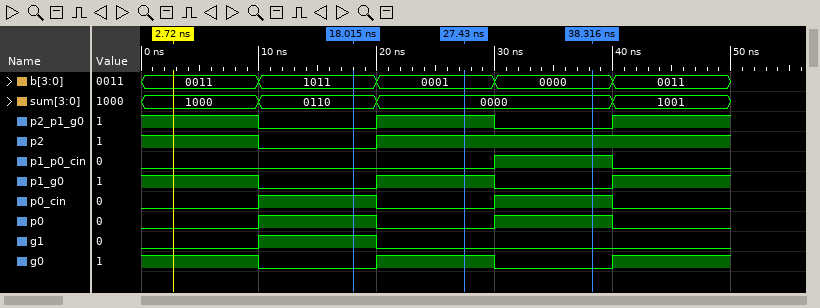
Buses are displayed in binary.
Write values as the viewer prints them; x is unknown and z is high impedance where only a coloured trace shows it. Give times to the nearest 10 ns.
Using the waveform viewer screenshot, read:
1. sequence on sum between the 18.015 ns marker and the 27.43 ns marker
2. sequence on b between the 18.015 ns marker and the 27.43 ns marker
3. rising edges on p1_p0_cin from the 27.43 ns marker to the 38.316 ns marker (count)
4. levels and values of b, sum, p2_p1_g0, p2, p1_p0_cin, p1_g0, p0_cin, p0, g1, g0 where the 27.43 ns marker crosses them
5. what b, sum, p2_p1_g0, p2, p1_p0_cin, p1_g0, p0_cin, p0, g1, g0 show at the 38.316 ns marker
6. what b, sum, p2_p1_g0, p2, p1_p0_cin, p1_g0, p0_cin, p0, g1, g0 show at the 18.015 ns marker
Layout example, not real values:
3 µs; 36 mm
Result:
0110, 0000; 1011, 0001; 1; b=0001, sum=0000, p2_p1_g0=1, p2=1, p1_p0_cin=0, p1_g0=1, p0_cin=0, p0=0, g1=0, g0=1; b=0000, sum=0000, p2_p1_g0=0, p2=1, p1_p0_cin=1, p1_g0=0, p0_cin=1, p0=1, g1=0, g0=0; b=1011, sum=0110, p2_p1_g0=0, p2=0, p1_p0_cin=0, p1_g0=0, p0_cin=1, p0=1, g1=1, g0=0
